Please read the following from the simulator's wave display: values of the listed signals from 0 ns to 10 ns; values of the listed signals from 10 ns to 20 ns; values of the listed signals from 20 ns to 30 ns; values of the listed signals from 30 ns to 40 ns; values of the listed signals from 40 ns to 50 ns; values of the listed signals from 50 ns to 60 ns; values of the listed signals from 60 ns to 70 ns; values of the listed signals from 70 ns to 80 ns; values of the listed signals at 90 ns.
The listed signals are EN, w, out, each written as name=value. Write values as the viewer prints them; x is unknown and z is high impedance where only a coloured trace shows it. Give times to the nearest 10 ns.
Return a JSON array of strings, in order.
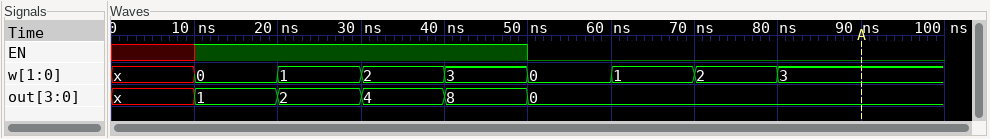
["EN=x, w=x, out=x", "EN=1, w=0, out=1", "EN=1, w=1, out=2", "EN=1, w=2, out=4", "EN=1, w=3, out=8", "EN=0, w=0, out=0", "EN=0, w=1, out=0", "EN=0, w=2, out=0", "EN=0, w=3, out=0"]
